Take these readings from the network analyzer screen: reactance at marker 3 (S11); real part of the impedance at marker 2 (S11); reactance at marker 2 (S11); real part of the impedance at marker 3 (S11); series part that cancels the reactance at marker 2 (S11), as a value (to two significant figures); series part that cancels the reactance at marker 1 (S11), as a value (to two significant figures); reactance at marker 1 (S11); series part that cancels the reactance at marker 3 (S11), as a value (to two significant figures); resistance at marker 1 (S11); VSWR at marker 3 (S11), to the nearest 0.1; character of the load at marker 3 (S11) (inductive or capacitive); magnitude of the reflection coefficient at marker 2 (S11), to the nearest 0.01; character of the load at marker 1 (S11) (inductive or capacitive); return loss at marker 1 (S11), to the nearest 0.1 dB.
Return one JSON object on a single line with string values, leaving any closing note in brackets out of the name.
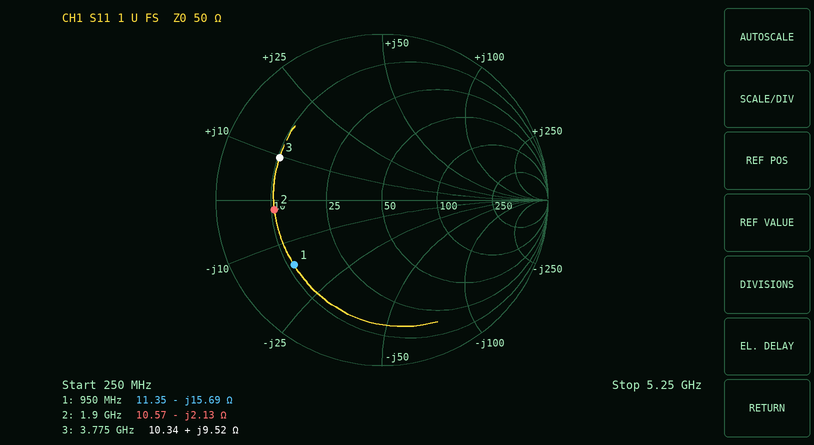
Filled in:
{"reactance at marker 3": "+9.52 Ω", "real part of the impedance at marker 2": "10.57 Ω", "reactance at marker 2": "-2.13 Ω", "real part of the impedance at marker 3": "10.34 Ω", "series part that cancels the reactance at marker 2 (S11), as a value": "180 pH", "series part that cancels the reactance at marker 1 (S11), as a value": "2.6 nH", "reactance at marker 1": "-15.69 Ω", "series part that cancels the reactance at marker 3 (S11), as a value": "4.4 pF", "resistance at marker 1": "11.35 Ω", "VSWR at marker 3 (S11), to the nearest 0.1": "5.0", "character of the load at marker 3 (S11)": "inductive", "magnitude of the reflection coefficient at marker 2 (S11), to the nearest 0.01": "0.65", "character of the load at marker 1 (S11)": "capacitive", "return loss at marker 1 (S11), to the nearest 0.1 dB": "3.6 dB"}
